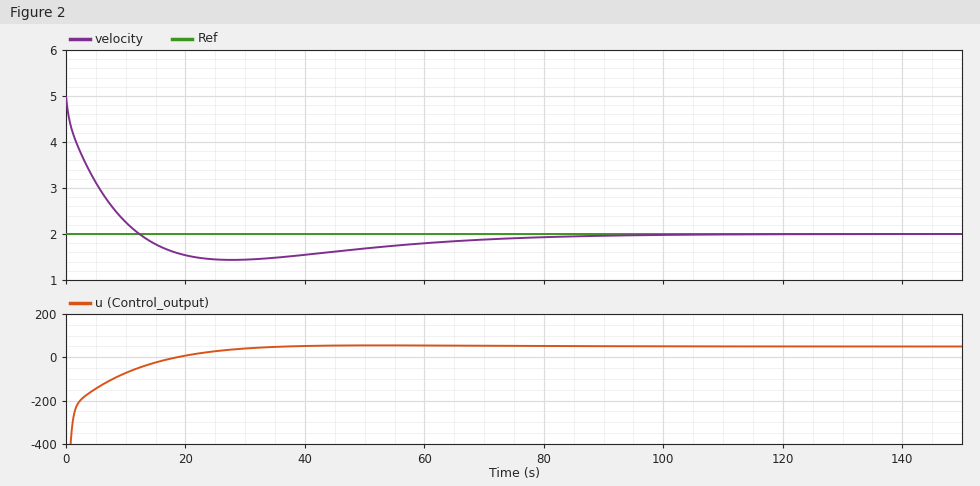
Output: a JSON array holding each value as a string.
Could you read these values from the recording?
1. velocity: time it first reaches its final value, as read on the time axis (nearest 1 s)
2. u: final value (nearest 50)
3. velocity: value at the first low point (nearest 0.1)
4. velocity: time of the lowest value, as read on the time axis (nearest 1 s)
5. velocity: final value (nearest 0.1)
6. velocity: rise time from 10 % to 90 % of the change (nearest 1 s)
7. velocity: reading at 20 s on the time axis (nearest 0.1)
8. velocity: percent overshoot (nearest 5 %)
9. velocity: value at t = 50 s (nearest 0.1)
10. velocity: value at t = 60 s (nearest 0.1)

["12 s", "50", "1.4", "28 s", "2.0", "9 s", "1.5", "20 %", "1.7", "1.8"]
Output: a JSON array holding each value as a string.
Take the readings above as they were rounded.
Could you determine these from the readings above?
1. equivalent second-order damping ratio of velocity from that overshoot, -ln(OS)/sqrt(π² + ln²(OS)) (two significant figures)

["0.46"]
